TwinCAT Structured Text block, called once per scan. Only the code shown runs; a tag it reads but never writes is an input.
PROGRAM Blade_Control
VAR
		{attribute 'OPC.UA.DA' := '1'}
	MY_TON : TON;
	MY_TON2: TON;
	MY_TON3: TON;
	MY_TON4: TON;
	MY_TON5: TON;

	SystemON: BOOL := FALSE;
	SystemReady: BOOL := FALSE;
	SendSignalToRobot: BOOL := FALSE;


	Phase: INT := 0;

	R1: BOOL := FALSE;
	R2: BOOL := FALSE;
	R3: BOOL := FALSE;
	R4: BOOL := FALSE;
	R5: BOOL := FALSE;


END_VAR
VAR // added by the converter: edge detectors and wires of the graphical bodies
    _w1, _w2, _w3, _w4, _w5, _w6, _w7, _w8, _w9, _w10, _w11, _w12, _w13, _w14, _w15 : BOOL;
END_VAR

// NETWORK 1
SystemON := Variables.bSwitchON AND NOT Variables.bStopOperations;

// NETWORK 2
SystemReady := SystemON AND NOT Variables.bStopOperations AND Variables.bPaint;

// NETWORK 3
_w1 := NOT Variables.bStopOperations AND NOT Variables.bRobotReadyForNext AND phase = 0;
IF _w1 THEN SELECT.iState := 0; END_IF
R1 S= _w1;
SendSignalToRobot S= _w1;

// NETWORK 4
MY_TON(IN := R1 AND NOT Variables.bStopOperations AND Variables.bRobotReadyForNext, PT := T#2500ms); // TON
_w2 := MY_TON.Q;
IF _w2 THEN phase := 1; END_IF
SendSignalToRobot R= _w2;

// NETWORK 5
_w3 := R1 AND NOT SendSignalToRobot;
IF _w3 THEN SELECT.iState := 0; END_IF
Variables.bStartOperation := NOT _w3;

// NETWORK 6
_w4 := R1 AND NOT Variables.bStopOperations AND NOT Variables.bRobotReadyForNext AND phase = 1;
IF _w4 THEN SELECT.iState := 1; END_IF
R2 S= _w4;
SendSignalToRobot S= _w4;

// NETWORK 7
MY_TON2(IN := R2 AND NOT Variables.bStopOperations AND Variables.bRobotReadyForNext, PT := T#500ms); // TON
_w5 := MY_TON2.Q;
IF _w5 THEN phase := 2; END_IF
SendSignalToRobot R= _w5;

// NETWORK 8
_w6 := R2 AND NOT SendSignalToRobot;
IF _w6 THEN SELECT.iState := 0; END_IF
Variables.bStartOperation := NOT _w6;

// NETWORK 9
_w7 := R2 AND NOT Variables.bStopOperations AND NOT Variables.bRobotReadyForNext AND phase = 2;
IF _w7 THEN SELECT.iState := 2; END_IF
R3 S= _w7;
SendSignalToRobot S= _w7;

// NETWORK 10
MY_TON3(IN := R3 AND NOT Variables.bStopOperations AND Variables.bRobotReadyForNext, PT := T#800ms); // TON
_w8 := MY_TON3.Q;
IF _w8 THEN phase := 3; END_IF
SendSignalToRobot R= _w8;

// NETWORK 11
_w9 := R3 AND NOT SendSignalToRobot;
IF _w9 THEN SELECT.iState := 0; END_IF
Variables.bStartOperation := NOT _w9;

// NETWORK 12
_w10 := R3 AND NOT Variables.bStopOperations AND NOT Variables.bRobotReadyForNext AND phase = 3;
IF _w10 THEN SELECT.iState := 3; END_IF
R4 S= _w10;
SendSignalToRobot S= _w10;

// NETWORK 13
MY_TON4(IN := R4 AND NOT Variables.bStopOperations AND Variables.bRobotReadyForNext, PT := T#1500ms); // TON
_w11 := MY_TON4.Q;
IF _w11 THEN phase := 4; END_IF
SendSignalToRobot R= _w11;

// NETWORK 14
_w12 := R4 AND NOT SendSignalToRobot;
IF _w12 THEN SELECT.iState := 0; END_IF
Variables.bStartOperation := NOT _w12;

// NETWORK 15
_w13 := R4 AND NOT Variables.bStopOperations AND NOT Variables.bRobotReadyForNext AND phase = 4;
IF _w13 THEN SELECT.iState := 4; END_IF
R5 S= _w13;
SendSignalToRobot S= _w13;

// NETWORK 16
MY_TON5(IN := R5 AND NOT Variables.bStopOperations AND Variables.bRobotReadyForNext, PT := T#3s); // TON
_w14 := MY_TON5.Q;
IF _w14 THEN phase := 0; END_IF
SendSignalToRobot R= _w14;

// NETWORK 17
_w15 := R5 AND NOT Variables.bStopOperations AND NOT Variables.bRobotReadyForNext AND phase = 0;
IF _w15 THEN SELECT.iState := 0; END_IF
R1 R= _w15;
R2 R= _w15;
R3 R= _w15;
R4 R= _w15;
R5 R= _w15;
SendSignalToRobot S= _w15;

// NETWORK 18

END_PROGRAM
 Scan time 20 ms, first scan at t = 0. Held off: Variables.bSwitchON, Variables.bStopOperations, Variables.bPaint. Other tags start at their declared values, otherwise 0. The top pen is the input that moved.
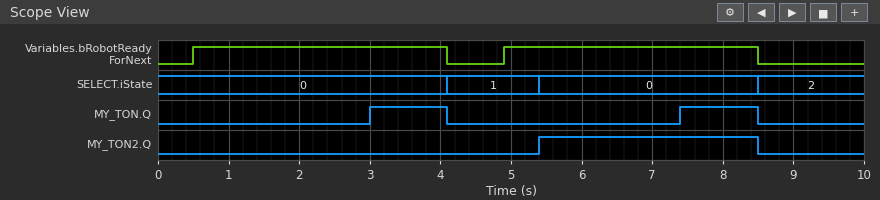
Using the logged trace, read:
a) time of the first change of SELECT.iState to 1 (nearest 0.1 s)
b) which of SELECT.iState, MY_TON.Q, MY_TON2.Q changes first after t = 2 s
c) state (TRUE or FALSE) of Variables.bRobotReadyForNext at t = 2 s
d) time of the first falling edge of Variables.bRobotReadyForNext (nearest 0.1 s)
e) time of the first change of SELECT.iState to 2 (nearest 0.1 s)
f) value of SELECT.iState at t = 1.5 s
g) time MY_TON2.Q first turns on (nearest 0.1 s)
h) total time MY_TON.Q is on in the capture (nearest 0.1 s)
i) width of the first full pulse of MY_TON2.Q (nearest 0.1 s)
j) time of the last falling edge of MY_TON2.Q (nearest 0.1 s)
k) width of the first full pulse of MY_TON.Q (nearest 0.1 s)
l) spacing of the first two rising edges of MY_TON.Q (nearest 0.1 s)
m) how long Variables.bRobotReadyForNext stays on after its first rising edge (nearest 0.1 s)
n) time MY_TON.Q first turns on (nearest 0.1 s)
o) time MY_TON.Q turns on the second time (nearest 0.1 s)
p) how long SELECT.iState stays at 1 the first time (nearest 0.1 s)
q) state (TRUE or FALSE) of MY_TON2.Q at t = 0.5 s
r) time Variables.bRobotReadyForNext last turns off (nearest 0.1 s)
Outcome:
4.1 s
MY_TON.Q
TRUE
4.1 s
8.5 s
0
5.4 s
2.2 s
3.1 s
8.5 s
1.1 s
4.4 s
3.6 s
3.0 s
7.4 s
1.3 s
FALSE
8.5 s
